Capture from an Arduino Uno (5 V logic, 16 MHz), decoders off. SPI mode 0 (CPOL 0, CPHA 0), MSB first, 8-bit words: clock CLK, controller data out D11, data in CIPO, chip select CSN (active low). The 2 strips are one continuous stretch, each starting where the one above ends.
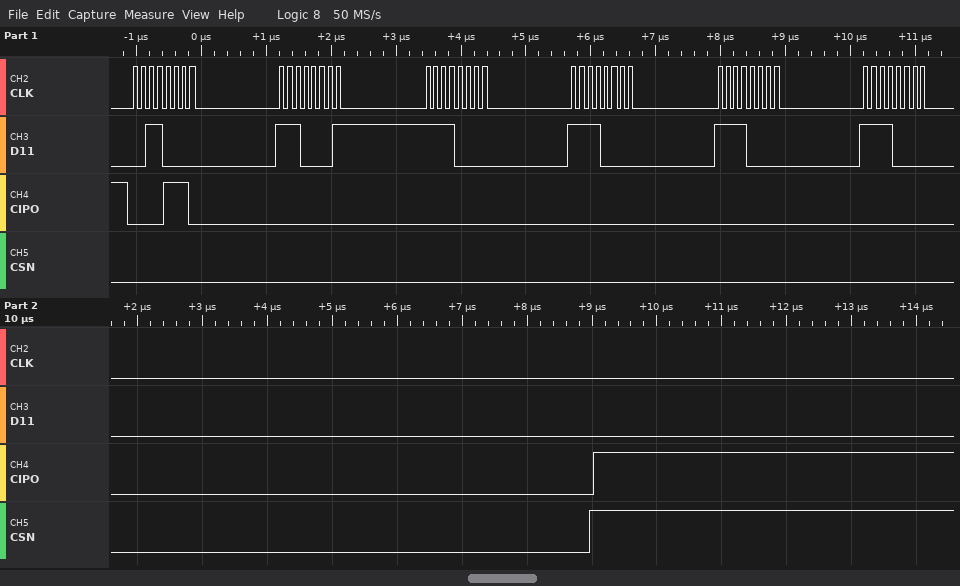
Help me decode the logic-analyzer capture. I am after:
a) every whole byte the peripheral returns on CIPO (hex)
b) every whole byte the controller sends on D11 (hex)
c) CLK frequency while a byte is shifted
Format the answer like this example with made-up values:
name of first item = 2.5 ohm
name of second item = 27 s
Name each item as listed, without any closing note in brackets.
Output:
every whole byte the peripheral returns on CIPO = 0E 00 00 00 00 00
every whole byte the controller sends on D11 = 30 E1 F0 F0 F0 F0
CLK frequency while a byte is shifted = 8 MHz
